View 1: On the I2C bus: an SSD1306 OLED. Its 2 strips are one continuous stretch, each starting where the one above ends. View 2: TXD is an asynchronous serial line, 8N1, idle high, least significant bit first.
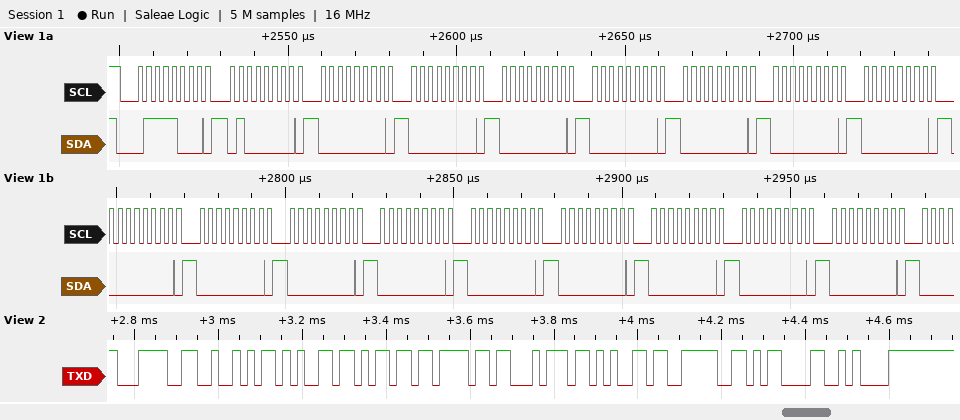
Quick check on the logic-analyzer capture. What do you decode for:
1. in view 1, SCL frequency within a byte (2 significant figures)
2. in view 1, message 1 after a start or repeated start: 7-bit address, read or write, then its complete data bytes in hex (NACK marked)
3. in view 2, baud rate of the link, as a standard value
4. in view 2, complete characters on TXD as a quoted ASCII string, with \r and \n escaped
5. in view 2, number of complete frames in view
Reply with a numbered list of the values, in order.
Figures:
1. 400 kHz
2. 0x3C write: 40 00 00 00 00 00 00 00 00 00 00 00 00 00 00 00 00
3. 57600 baud
4. "<Remote>\r\n"
5. 10
